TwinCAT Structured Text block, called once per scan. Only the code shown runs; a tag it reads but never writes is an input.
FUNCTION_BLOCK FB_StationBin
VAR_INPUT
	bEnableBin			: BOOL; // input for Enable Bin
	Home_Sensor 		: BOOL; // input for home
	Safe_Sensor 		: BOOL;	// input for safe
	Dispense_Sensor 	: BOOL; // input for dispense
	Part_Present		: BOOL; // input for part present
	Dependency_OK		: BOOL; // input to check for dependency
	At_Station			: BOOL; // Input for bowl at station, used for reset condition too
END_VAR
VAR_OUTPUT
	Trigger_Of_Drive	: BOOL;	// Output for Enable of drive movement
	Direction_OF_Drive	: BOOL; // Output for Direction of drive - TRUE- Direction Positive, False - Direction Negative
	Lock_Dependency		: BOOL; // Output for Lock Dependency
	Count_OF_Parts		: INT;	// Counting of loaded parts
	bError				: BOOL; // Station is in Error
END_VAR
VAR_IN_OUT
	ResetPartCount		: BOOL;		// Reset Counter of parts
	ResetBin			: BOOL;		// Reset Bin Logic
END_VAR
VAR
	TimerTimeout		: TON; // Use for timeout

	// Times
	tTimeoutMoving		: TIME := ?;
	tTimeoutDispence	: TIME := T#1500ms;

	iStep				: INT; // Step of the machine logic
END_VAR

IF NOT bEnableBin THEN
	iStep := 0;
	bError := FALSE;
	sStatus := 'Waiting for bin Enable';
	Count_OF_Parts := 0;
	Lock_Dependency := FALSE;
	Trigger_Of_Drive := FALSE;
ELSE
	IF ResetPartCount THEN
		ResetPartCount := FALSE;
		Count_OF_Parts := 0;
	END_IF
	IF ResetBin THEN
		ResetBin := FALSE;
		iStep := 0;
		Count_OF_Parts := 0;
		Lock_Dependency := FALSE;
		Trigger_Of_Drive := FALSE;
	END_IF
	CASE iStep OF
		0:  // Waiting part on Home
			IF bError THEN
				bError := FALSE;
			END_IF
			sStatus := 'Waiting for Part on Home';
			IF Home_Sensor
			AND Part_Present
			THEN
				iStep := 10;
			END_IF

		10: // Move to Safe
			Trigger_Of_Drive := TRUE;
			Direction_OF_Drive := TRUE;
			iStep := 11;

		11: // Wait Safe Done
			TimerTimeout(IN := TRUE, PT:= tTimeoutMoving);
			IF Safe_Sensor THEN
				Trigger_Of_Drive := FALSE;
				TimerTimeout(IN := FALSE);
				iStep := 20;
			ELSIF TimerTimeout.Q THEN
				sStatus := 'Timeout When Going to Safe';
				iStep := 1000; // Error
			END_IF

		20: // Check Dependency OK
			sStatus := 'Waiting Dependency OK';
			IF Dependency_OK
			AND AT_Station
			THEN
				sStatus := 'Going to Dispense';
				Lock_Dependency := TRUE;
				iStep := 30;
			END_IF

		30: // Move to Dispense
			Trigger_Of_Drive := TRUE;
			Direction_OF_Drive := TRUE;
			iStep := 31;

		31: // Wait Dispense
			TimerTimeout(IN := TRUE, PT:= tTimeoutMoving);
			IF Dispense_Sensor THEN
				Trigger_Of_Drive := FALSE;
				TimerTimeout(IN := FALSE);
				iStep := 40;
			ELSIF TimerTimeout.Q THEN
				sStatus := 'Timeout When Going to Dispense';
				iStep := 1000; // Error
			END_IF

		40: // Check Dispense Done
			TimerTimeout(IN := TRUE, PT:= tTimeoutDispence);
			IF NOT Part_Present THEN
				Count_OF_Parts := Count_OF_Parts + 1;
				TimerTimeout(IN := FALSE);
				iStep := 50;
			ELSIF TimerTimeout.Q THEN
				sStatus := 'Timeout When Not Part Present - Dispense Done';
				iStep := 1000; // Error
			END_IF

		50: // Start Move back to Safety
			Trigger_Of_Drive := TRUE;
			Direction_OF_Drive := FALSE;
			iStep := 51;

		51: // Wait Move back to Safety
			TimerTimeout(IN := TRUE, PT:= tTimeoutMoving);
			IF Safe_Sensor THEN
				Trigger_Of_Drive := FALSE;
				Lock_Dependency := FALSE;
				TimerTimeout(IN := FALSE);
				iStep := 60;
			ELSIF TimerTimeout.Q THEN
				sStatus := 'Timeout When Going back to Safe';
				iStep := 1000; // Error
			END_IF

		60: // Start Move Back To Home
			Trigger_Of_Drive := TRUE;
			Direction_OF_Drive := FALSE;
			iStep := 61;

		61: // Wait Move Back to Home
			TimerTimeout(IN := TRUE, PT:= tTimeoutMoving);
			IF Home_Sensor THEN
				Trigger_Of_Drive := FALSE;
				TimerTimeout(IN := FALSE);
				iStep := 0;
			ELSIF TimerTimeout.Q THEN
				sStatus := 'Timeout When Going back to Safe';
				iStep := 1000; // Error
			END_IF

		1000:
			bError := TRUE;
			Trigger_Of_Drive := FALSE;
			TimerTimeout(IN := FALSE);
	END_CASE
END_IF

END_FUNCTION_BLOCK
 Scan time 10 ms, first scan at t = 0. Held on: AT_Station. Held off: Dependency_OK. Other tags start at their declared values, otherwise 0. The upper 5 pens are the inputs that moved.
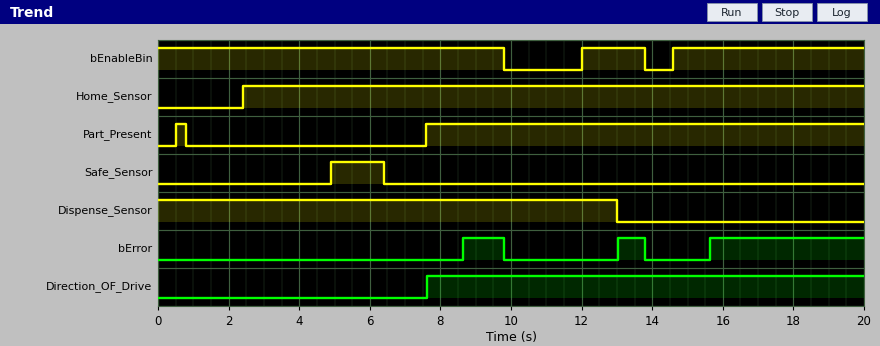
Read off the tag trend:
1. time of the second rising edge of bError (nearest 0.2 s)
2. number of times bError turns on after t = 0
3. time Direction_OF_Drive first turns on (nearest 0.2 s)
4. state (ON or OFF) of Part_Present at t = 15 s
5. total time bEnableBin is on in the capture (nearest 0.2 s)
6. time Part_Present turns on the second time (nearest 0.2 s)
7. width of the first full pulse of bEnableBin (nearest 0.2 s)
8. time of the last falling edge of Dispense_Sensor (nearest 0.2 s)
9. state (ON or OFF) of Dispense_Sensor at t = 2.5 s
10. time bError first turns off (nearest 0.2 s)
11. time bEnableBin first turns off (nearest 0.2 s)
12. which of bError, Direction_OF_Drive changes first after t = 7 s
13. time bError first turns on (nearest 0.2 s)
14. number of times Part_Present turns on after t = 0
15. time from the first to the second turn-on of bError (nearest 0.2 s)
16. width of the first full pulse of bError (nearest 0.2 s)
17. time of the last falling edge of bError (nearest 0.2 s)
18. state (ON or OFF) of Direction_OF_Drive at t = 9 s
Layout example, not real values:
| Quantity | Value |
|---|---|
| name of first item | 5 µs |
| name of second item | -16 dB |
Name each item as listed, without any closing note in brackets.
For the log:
| Quantity | Value |
|---|---|
| time of the second rising edge of bError | 13.0 s |
| number of times bError turns on after t = 0 | 3 |
| time Direction_OF_Drive first turns on | 7.6 s |
| state (ON or OFF) of Part_Present at t = 15 s | ON |
| total time bEnableBin is on in the capture | 17.0 s |
| time Part_Present turns on the second time | 7.6 s |
| width of the first full pulse of bEnableBin | 1.8 s |
| time of the last falling edge of Dispense_Sensor | 13.0 s |
| state (ON or OFF) of Dispense_Sensor at t = 2.5 s | ON |
| time bError first turns off | 9.8 s |
| time bEnableBin first turns off | 9.8 s |
| which of bError, Direction_OF_Drive changes first after t = 7 s | Direction_OF_Drive |
| time bError first turns on | 8.6 s |
| number of times Part_Present turns on after t = 0 | 2 |
| time from the first to the second turn-on of bError | 4.4 s |
| width of the first full pulse of bError | 1.2 s |
| time of the last falling edge of bError | 13.8 s |
| state (ON or OFF) of Direction_OF_Drive at t = 9 s | ON |
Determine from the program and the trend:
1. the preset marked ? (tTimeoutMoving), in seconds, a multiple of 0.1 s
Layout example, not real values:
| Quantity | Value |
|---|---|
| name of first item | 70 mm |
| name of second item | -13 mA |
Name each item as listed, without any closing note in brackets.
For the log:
| Quantity | Value |
|---|---|
| the preset marked ? (tTimeoutMoving), in seconds, a multiple of 0.1 s | 1.0 s |
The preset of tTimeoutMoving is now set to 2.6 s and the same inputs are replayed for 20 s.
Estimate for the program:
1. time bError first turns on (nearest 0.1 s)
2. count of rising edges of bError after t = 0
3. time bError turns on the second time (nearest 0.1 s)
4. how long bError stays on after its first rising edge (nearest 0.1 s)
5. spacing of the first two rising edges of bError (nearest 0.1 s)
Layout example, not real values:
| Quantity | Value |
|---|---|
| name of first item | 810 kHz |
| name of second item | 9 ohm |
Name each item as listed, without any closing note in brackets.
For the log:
| Quantity | Value |
|---|---|
| time bError first turns on | 12.0 s |
| count of rising edges of bError after t = 0 | 2 |
| time bError turns on the second time | 17.2 s |
| how long bError stays on after its first rising edge | 1.8 s |
| spacing of the first two rising edges of bError | 5.2 s |
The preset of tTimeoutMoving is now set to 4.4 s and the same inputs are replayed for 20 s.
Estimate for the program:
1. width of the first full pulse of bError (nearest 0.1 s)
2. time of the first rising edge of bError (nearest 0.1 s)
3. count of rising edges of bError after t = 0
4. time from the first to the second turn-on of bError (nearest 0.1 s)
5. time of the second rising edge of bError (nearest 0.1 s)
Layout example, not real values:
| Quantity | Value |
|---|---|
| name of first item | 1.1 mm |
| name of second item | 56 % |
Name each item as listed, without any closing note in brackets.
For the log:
| Quantity | Value |
|---|---|
| width of the first full pulse of bError | 1.8 s |
| time of the first rising edge of bError | 12.0 s |
| count of rising edges of bError after t = 0 | 2 |
| time from the first to the second turn-on of bError | 7.0 s |
| time of the second rising edge of bError | 19.0 s |
